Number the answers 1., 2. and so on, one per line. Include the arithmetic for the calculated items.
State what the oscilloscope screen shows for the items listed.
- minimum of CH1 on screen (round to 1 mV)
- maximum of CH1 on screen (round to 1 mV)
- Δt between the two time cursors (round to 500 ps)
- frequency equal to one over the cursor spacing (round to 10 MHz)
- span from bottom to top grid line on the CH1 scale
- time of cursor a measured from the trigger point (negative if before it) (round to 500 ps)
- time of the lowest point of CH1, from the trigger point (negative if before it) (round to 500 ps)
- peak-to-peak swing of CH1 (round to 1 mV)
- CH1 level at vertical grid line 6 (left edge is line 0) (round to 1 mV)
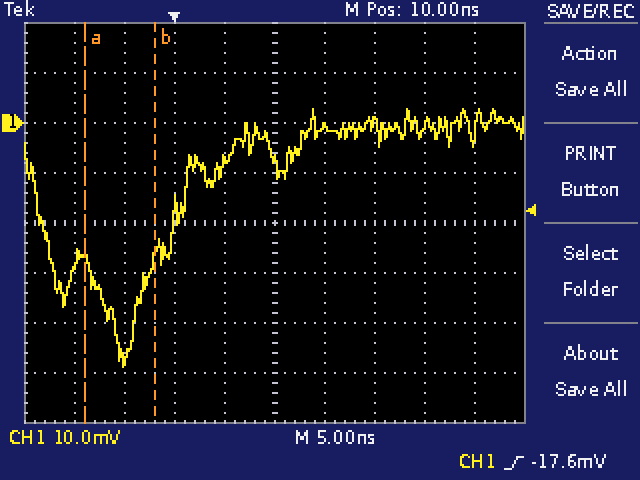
1. -49 mV
2. 3 mV
3. 7.0 ns
4. 1 / 7.0 ns ≈ 140 MHz
5. 80 mV
6. -9.0 ns
7. -5.0 ns
8. 3 mV − (-49 mV) = 52 mV
9. -1 mV
